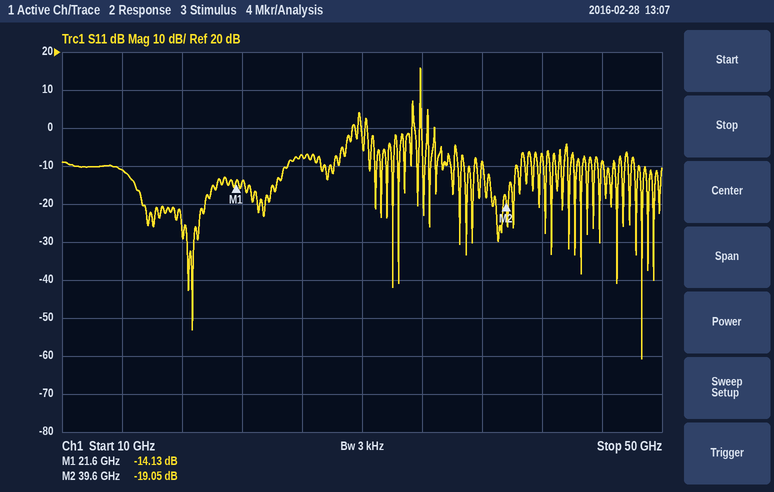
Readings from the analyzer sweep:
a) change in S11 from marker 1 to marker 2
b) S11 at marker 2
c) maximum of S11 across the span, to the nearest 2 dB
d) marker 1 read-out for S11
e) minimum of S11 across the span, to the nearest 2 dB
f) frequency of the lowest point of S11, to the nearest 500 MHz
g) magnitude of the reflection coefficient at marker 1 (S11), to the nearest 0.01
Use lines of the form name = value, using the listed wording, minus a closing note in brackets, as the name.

change in S11 from marker 1 to marker 2 = -4.92 dB
S11 at marker 2 = -19.05 dB
maximum of S11 across the span, to the nearest 2 dB = 16 dB
marker 1 read-out for S11 = -14.13 dB
minimum of S11 across the span, to the nearest 2 dB = -60 dB
frequency of the lowest point of S11, to the nearest 500 MHz = 48.5 GHz
magnitude of the reflection coefficient at marker 1 (S11), to the nearest 0.01 = 0.20
